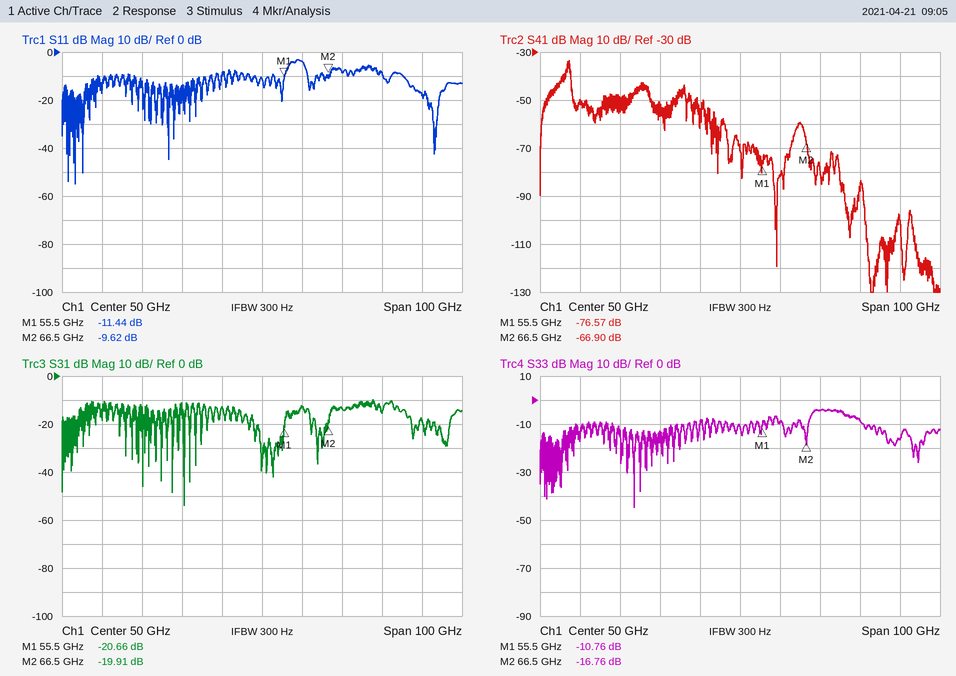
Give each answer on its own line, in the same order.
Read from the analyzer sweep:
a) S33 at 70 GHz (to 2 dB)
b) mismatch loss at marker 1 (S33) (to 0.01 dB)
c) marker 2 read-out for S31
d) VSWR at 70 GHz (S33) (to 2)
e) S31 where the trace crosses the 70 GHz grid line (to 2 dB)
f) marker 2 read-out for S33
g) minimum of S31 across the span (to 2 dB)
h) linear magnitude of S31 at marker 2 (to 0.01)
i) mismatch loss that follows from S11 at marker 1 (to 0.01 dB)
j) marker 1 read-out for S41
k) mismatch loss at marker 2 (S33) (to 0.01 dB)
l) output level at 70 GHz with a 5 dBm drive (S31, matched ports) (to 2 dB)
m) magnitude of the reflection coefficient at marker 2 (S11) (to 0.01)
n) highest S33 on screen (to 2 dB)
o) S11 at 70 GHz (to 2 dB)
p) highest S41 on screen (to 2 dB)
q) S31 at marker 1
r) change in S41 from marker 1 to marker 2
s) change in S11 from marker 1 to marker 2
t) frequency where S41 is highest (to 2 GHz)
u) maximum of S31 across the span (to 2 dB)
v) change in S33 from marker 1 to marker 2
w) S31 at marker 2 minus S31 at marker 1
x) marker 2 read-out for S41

-4 dB
0.38 dB
-19.91 dB
4
-14 dB
-16.76 dB
-54 dB
0.10
0.32 dB
-76.57 dB
0.09 dB
-8 dBm
0.33
-4 dB
-8 dB
-34 dB
-20.66 dB
9.67 dB
1.82 dB
8 GHz
-10 dB
-6.00 dB
0.75 dB
-66.90 dB
